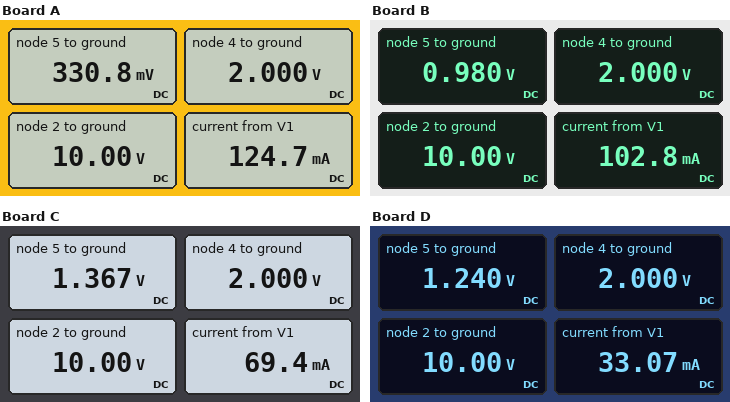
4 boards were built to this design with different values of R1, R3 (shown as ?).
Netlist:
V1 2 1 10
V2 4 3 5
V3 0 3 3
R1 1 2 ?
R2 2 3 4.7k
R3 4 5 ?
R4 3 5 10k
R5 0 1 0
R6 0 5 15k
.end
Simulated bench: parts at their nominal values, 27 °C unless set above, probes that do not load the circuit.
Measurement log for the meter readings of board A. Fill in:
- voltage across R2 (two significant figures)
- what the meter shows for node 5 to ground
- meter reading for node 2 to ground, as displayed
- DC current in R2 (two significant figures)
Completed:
13 V
330.8 mV
10.00 V
2.8 mA
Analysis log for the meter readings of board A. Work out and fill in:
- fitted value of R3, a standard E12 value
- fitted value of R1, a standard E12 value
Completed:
4.7 kΩ
82 Ω
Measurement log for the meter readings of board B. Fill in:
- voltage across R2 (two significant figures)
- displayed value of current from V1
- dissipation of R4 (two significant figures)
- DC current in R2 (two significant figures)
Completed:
13 V
102.8 mA
1.6 mW
2.8 mA
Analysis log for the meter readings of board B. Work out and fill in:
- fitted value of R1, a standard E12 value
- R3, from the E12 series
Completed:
100 Ω
2.2 kΩ
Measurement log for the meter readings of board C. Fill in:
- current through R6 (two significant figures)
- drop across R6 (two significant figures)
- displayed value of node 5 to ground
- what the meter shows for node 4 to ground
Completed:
91 µA
1.4 V
1.367 V
2.000 V
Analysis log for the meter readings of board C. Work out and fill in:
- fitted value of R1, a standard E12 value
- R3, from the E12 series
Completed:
150 Ω
1.2 kΩ
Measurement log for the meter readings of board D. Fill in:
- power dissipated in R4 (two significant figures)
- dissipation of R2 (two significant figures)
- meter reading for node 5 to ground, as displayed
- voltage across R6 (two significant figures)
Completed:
1.8 mW
36 mW
1.240 V
1.2 V
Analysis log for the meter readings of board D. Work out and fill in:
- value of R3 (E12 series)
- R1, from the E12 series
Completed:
1.5 kΩ
330 Ω
